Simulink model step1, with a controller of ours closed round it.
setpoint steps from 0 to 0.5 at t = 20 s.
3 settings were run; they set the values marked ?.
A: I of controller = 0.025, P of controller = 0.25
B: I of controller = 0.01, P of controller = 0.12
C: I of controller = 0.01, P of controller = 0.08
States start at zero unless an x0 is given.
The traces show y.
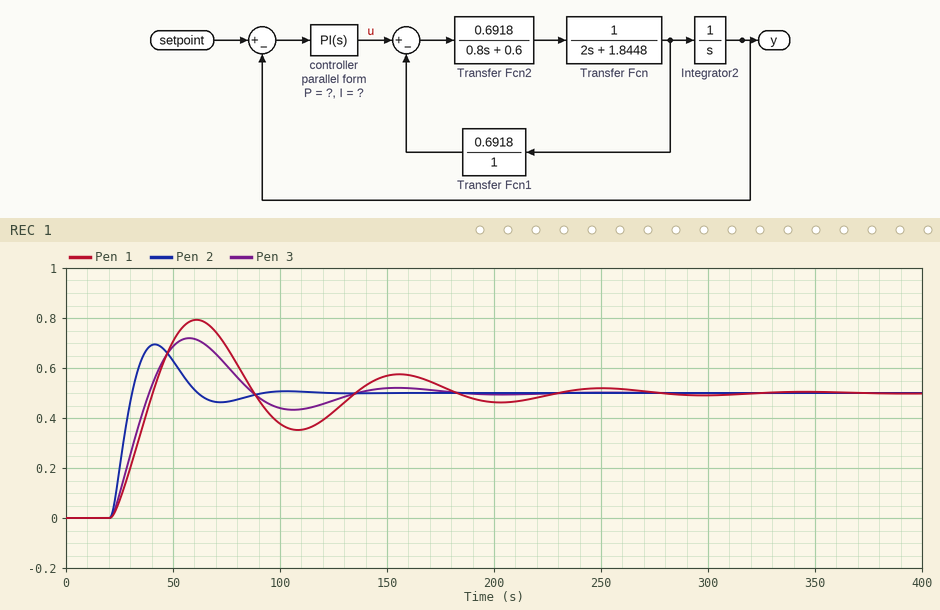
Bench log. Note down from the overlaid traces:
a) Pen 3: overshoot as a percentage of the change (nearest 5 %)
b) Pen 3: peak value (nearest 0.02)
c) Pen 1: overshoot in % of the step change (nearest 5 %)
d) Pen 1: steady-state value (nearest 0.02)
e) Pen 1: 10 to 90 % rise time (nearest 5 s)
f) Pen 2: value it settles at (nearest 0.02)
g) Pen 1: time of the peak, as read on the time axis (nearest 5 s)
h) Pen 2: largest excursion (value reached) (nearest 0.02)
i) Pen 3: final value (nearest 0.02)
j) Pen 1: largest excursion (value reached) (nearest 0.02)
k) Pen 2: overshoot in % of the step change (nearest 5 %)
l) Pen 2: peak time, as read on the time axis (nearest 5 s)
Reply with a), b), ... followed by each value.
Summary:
a) 45 %
b) 0.72
c) 60 %
d) 0.50
e) 15 s
f) 0.50
g) 60 s
h) 0.70
i) 0.50
j) 0.80
k) 40 %
l) 40 s
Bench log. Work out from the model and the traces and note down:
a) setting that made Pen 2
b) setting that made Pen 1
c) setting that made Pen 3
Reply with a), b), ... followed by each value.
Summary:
a) A
b) C
c) B
